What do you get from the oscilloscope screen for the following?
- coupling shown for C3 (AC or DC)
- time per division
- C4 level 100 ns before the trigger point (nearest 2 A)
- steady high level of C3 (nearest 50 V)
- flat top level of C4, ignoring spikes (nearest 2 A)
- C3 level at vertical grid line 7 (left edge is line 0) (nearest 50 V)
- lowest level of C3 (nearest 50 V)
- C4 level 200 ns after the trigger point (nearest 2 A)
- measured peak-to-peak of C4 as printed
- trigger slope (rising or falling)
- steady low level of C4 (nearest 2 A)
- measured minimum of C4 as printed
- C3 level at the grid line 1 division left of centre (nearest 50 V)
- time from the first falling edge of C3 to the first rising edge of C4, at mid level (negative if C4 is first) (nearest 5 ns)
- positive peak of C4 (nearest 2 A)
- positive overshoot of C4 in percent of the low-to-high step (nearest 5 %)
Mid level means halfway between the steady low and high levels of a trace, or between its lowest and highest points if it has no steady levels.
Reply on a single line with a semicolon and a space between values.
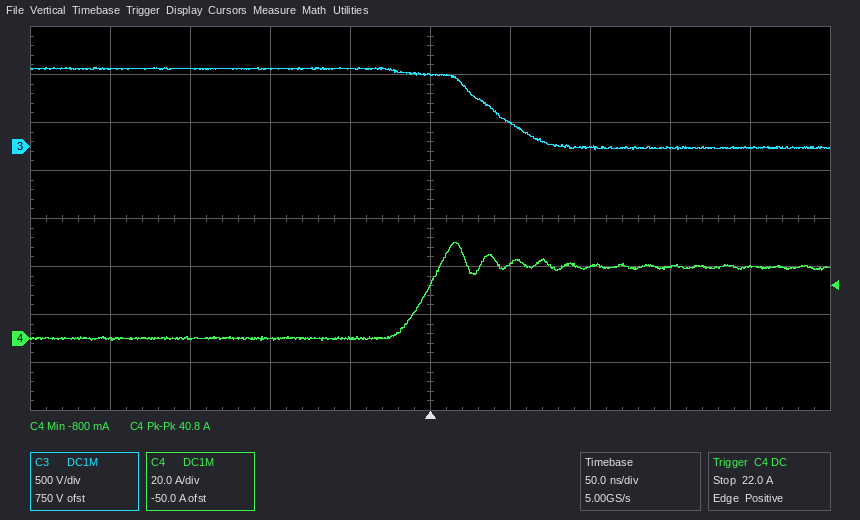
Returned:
DC; 50 ns; 0 A; 800 V; 30 A; 0 V; -50 V; 30 A; 40.8 A; rising; 0 A; -800 mA; 800 V; -45 ns; 40 A; 35 %
